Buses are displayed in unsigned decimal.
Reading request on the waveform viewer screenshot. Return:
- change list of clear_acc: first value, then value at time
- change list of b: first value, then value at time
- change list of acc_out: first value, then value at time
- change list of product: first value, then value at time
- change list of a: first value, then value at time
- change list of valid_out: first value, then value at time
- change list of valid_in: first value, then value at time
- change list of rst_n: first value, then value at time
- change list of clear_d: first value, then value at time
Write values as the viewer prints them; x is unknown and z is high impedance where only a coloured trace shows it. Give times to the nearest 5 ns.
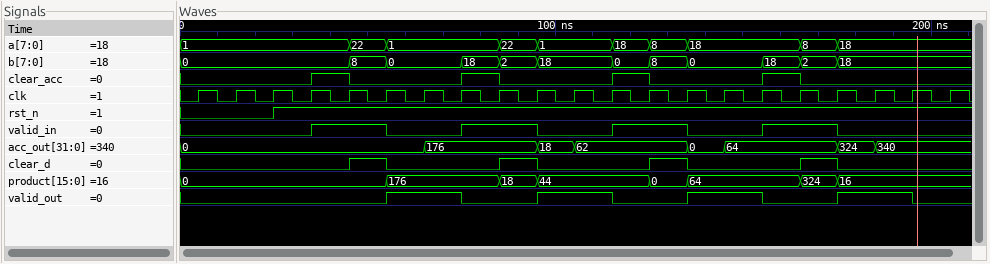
0, 1 at 35 ns, 0 at 45 ns, 1 at 75 ns, 0 at 85 ns, 1 at 115 ns, 0 at 125 ns, 1 at 155 ns, 0 at 165 ns
0, 8 at 45 ns, 0 at 55 ns, 18 at 75 ns, 2 at 85 ns, 18 at 95 ns, 0 at 115 ns, 8 at 125 ns, 0 at 135 ns, 18 at 155 ns, 2 at 165 ns, 18 at 175 ns
0, 176 at 65 ns, 18 at 95 ns, 62 at 105 ns, 0 at 135 ns, 64 at 145 ns, 324 at 175 ns, 340 at 185 ns
0, 176 at 55 ns, 18 at 85 ns, 44 at 95 ns, 0 at 125 ns, 64 at 135 ns, 324 at 165 ns, 16 at 175 ns
1, 22 at 45 ns, 1 at 55 ns, 22 at 85 ns, 1 at 95 ns, 18 at 115 ns, 8 at 125 ns, 18 at 135 ns, 8 at 165 ns, 18 at 175 ns
0, 1 at 55 ns, 0 at 75 ns, 1 at 95 ns, 0 at 115 ns, 1 at 135 ns, 0 at 155 ns, 1 at 175 ns, 0 at 195 ns
0, 1 at 35 ns, 0 at 55 ns, 1 at 75 ns, 0 at 95 ns, 1 at 115 ns, 0 at 135 ns, 1 at 155 ns, 0 at 175 ns
0, 1 at 25 ns
0, 1 at 45 ns, 0 at 55 ns, 1 at 85 ns, 0 at 95 ns, 1 at 125 ns, 0 at 135 ns, 1 at 165 ns, 0 at 175 ns
